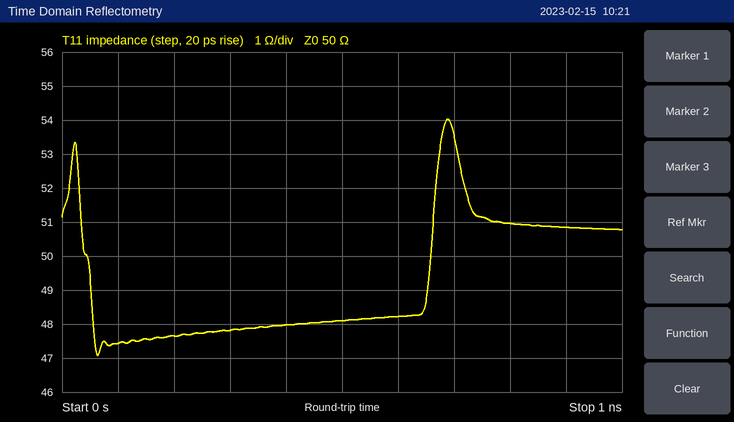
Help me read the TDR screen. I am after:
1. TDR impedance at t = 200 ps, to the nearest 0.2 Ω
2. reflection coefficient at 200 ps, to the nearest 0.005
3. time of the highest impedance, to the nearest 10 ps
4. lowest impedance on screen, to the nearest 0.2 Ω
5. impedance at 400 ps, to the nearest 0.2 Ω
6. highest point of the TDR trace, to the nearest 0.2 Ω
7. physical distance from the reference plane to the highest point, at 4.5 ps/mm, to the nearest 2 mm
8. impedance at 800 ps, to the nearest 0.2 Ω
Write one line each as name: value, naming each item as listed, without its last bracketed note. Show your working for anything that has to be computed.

TDR impedance at t = 200 ps, to the nearest 0.2 Ω: 47.6 Ω
reflection coefficient at 200 ps, to the nearest 0.005: (47.6 − 50)/(47.6 + 50) ≈ -0.025
time of the highest impedance, to the nearest 10 ps: 690 ps
lowest impedance on screen, to the nearest 0.2 Ω: 47.0 Ω
impedance at 400 ps, to the nearest 0.2 Ω: 48.0 Ω
highest point of the TDR trace, to the nearest 0.2 Ω: 54.0 Ω
physical distance from the reference plane to the highest point, at 4.5 ps/mm, to the nearest 2 mm: 690 ps / 2 / 4.5 ps/mm ≈ 76.7 mm, so 76 mm to the nearest 2 mm
impedance at 800 ps, to the nearest 0.2 Ω: 51.0 Ω
